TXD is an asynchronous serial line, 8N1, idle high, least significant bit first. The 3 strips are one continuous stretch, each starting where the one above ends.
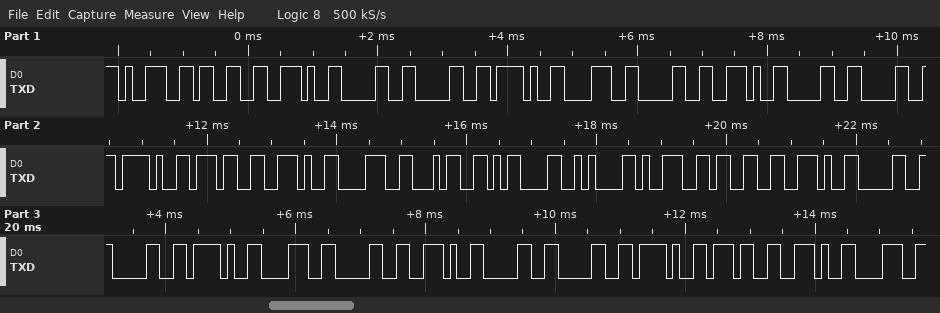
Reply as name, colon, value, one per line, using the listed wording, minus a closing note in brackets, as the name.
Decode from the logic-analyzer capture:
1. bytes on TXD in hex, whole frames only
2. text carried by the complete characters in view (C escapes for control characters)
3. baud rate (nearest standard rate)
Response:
bytes on TXD in hex, whole frames only: 39 33 2E 30 30 2F 38 30 2E 30 30 2F 37 2E 38 34 0D 0A 39 33 2E 30 30 2F 38 30 2E 30 30 2F 37 2E 38
text carried by the complete characters in view: "93.00/80.00/7.84\r\n93.00/80.00/7.8"
baud rate: 9600 baud
